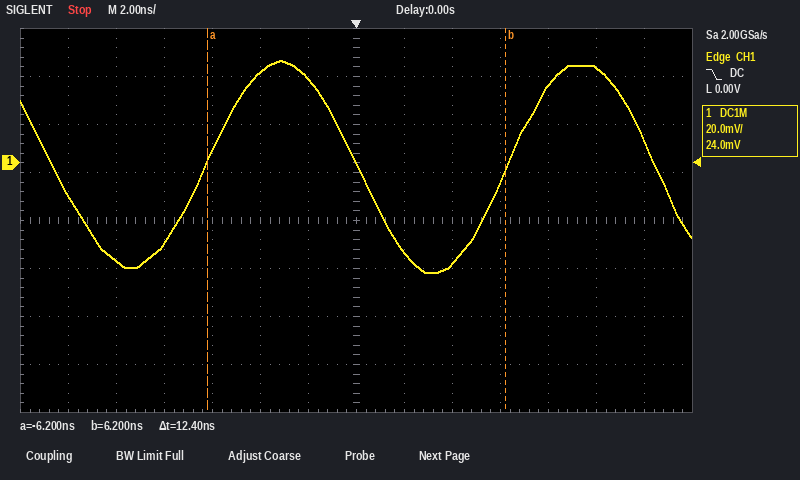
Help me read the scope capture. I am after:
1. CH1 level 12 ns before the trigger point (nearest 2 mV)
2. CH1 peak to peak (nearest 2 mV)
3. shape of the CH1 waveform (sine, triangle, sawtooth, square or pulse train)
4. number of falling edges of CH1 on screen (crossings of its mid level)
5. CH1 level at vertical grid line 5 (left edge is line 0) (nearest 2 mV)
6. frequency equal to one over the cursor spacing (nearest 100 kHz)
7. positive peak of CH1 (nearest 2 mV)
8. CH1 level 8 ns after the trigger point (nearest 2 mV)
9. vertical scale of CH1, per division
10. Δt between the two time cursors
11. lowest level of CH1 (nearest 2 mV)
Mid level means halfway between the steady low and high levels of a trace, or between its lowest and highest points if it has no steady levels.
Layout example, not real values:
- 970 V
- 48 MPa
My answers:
- -14 mV
- 88 mV
- sine
- 3
- 38 mV
- 80.6 MHz
- 42 mV
- 32 mV
- 20 mV
- 12.4 ns
- -46 mV
